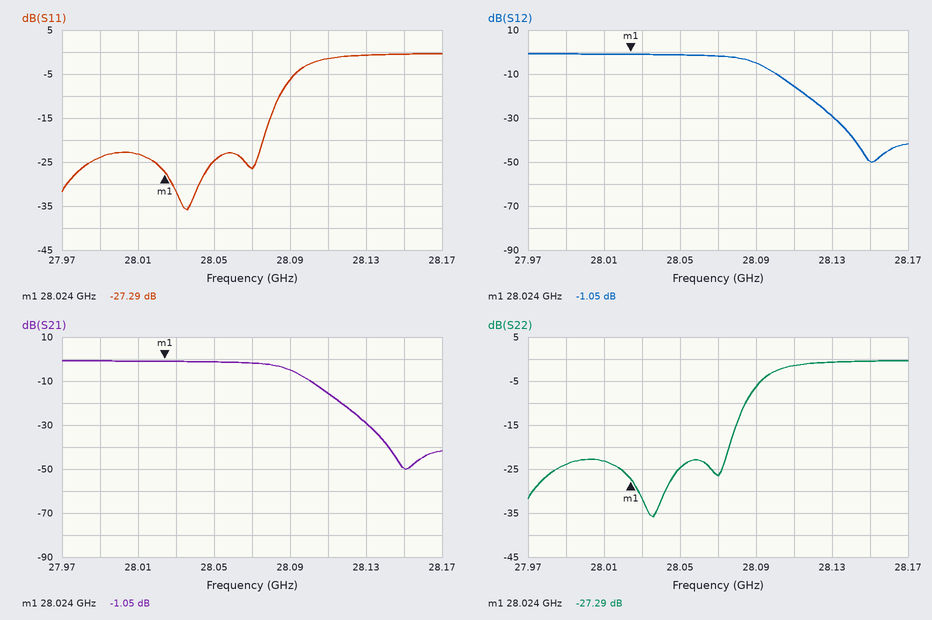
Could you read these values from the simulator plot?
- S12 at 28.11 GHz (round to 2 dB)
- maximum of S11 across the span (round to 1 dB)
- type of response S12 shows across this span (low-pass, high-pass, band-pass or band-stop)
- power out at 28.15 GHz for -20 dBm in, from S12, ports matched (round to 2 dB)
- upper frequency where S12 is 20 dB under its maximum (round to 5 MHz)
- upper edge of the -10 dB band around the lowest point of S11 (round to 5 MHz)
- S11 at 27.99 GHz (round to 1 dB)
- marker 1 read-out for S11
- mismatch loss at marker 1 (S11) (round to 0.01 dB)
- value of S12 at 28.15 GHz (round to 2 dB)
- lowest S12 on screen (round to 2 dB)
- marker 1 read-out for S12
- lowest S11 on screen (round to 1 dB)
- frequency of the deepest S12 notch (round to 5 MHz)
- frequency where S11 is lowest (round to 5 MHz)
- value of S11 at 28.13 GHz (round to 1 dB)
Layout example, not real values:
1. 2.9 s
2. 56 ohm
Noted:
1. -16 dB
2. 0 dB
3. low-pass
4. -70 dBm
5. 28.120 GHz
6. 28.085 GHz
7. -24 dB
8. -27.29 dB
9. 0.01 dB
10. -50 dB
11. -50 dB
12. -1.05 dB
13. -36 dB
14. 28.150 GHz
15. 28.035 GHz
16. -1 dB
